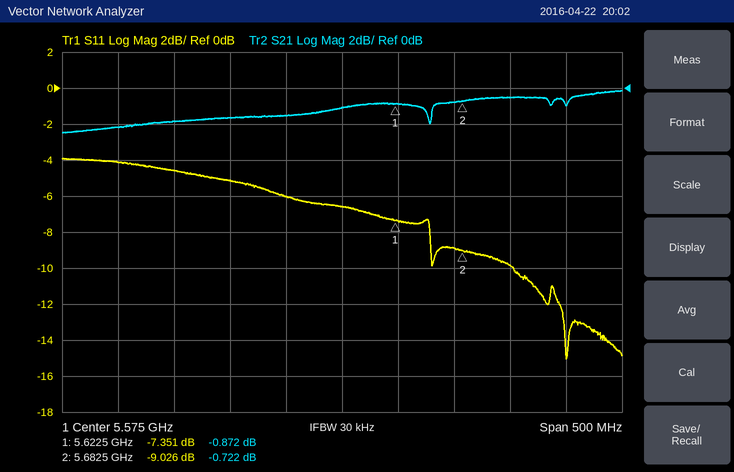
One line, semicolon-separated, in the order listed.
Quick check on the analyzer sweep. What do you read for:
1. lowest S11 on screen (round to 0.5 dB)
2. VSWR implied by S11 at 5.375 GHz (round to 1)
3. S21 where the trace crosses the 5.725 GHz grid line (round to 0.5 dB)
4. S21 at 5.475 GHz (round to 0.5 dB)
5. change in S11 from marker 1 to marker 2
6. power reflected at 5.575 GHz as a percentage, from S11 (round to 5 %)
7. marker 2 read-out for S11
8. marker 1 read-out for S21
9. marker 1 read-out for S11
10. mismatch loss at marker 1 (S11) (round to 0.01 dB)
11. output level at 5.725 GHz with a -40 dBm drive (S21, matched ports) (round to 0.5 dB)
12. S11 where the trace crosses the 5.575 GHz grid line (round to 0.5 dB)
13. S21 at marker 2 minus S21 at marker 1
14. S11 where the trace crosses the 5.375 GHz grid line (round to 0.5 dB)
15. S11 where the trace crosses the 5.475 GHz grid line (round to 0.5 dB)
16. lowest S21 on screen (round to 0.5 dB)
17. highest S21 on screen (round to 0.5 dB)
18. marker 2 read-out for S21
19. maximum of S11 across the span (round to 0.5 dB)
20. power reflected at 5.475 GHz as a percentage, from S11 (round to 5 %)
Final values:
-15.0 dB; 4; -0.5 dB; -1.5 dB; -1.675 dB; 20 %; -9.026 dB; -0.872 dB; -7.351 dB; 0.88 dB; -40.5 dBm; -6.5 dB; 0.150 dB; -4.0 dB; -5.0 dB; -2.5 dB; 0.0 dB; -0.722 dB; -4.0 dB; 30 %
